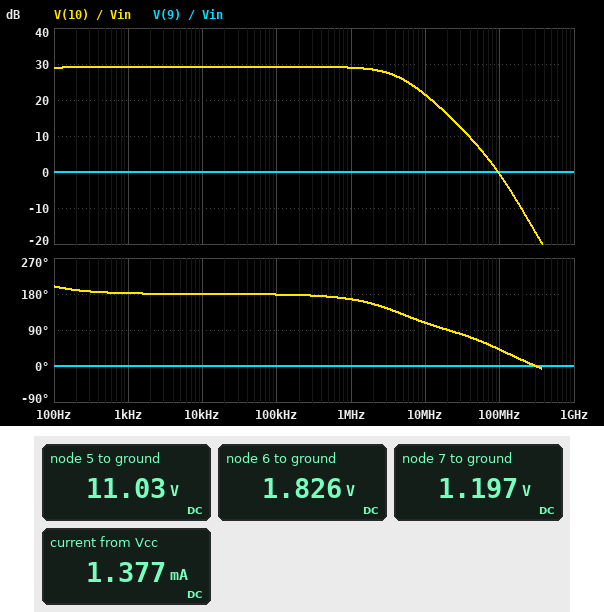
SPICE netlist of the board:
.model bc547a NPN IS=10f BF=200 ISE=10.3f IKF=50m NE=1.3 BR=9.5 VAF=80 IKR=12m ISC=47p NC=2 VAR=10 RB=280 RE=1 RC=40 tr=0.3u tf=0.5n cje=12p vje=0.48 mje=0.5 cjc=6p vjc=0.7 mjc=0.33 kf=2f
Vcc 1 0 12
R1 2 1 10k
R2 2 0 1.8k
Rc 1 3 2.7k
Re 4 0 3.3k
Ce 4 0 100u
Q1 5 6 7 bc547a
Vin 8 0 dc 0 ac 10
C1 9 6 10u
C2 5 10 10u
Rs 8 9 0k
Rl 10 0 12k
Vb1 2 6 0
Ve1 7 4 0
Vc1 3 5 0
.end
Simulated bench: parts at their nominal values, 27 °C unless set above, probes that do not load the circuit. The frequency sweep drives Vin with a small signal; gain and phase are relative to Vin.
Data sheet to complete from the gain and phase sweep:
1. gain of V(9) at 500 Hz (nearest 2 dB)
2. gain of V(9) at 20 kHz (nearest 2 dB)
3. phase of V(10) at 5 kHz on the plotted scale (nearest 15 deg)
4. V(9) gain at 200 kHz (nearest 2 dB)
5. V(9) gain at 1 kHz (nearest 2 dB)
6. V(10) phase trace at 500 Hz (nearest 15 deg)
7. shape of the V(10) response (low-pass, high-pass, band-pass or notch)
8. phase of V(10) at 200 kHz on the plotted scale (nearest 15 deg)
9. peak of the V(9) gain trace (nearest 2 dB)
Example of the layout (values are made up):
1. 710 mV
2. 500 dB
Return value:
1. 0 dB
2. 0 dB
3. 180 deg
4. 0 dB
5. 0 dB
6. 180 deg
7. low-pass
8. 180 deg
9. 0 dB
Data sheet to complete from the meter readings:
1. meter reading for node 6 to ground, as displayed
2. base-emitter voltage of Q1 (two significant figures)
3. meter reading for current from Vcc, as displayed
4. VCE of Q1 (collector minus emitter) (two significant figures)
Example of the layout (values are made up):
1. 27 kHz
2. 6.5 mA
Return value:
1. 1.826 V
2. 630 mV
3. 1.377 mA
4. 9.8 V
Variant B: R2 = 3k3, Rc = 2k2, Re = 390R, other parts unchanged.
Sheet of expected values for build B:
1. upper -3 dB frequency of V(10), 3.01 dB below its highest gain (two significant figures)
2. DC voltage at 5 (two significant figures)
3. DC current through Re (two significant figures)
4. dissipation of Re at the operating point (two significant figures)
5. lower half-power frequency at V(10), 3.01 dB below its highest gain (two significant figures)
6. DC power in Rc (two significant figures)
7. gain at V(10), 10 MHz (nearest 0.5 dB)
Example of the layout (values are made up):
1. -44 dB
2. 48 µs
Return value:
1. 75 kHz
2. 2.1 V
3. 4.7 mA
4. 8.5 mW
5. 60 Hz
6. 45 mW
7. -33.5 dB
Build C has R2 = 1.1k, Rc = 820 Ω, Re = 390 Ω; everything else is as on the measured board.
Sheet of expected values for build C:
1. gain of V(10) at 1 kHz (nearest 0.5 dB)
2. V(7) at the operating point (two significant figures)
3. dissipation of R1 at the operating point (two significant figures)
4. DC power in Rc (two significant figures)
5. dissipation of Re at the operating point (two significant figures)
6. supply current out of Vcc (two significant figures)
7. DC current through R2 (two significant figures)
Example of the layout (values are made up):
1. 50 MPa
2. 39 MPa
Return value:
1. 30.0 dB
2. 510 mV
3. 12 mW
4. 1.4 mW
5. 680 µW
6. 2.4 mA
7. 1.1 mA
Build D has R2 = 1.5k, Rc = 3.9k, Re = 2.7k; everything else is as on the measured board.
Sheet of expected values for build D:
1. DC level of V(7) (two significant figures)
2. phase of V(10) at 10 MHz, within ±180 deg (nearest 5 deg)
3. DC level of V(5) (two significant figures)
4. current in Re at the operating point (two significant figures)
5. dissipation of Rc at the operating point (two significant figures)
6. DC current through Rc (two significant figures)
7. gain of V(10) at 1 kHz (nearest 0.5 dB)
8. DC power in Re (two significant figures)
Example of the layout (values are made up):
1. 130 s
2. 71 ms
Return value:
1. 930 mV
2. 105 deg
3. 11 V
4. 350 µA
5. 460 µW
6. 340 µA
7. 31.5 dB
8. 320 µW
